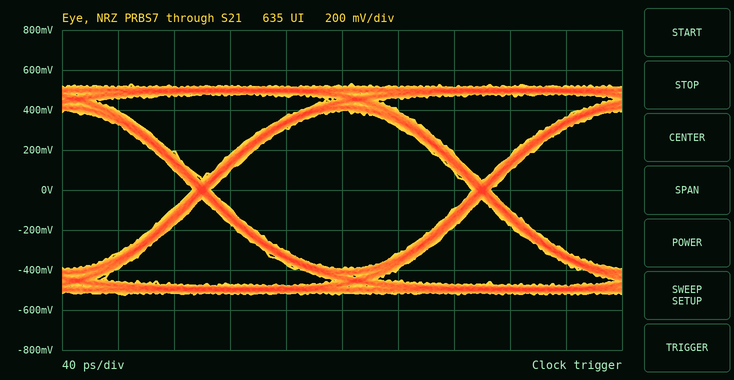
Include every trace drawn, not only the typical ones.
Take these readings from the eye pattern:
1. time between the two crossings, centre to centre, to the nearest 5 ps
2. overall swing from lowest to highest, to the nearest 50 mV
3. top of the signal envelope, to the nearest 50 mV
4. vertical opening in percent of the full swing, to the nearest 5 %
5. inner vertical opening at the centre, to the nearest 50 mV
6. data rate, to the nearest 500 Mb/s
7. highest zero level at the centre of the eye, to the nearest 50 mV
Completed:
200 ps
1.05 V
550 mV
75 %
800 mV
5.0 Gb/s
-400 mV
